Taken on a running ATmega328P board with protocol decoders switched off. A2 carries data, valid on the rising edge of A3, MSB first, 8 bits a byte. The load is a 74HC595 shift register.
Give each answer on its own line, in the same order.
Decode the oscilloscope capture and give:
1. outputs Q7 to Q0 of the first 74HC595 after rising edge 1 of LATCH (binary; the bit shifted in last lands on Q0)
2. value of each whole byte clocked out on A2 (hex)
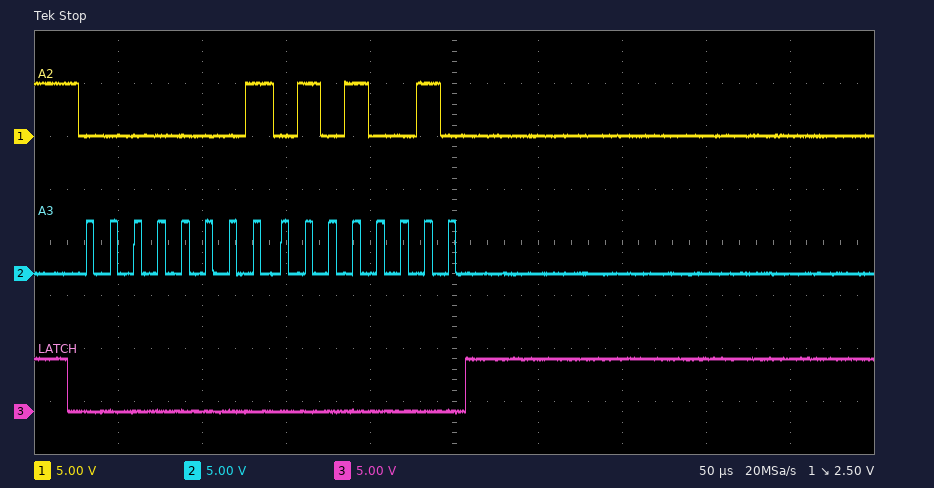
01010010
0x01 0x52
